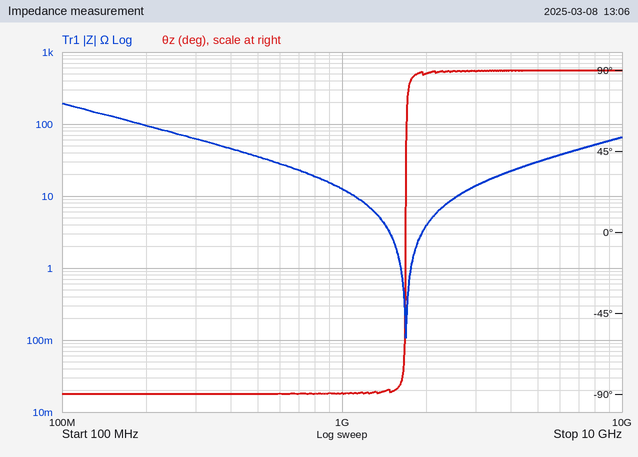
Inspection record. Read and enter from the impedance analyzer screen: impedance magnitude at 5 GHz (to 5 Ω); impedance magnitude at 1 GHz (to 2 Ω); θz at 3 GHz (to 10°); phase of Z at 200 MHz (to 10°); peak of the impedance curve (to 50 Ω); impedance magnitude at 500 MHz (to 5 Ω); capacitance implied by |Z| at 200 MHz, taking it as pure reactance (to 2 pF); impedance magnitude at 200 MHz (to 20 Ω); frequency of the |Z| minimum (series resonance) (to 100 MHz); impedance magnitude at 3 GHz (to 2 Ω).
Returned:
30 Ω
12 Ω
90°
-90°
200 Ω
35 Ω
8 pF
100 Ω
1.7 GHz
14 Ω
